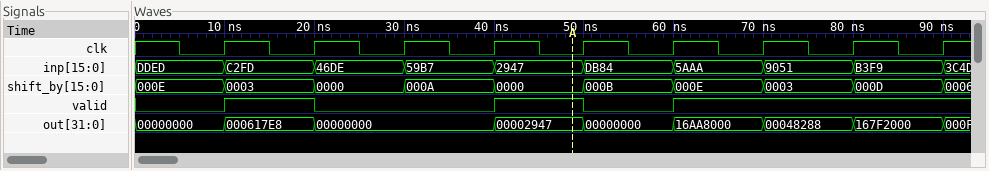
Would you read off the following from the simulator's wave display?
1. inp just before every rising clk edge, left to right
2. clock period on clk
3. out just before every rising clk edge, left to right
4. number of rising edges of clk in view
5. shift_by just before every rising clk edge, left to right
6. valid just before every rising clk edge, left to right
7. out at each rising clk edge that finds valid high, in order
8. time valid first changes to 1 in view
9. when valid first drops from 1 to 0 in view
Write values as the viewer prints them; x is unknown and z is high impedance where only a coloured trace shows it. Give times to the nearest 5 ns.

DDED, C2FD, 46DE, 59B7, 2947, DB84, 5AAA, 9051, B3F9
10 ns
00000000, 000617E8, 00000000, 00000000, 00002947, 00000000, 16AA8000, 00048288, 167F2000
9
000E, 0003, 0000, 000A, 0000, 000B, 000E, 0003, 000D
0 1 0 0 1 0 1 1 1
000617E8, 00002947, 16AA8000, 00048288, 167F2000
10 ns
20 ns
